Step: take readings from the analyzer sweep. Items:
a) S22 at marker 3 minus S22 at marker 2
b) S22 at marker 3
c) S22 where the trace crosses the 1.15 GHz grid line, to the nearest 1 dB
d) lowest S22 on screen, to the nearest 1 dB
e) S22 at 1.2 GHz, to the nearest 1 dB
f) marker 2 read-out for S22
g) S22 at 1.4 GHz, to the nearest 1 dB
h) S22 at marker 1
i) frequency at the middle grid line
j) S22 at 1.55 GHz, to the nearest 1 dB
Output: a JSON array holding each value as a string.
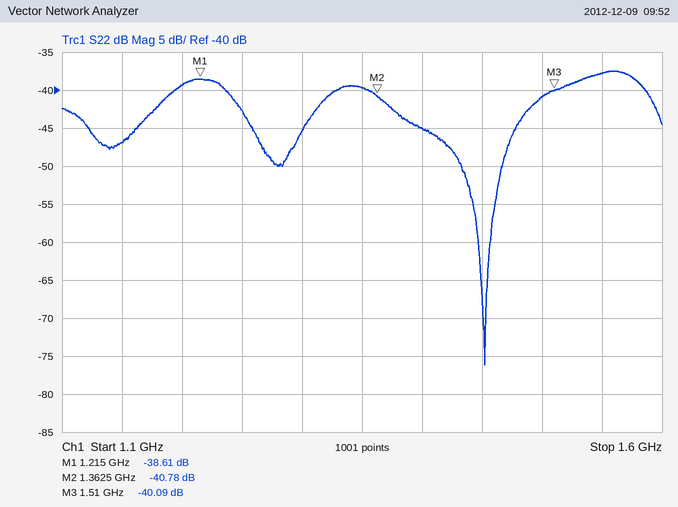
["0.69 dB", "-40.09 dB", "-47 dB", "-76 dB", "-39 dB", "-40.78 dB", "-45 dB", "-38.61 dB", "1.35 GHz", "-38 dB"]
